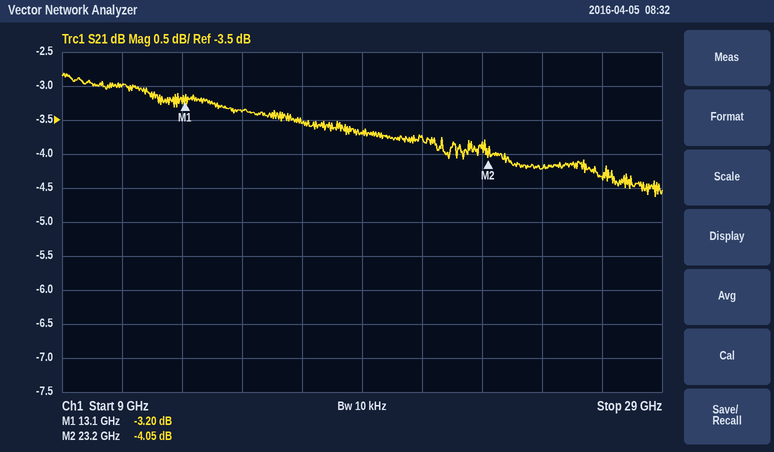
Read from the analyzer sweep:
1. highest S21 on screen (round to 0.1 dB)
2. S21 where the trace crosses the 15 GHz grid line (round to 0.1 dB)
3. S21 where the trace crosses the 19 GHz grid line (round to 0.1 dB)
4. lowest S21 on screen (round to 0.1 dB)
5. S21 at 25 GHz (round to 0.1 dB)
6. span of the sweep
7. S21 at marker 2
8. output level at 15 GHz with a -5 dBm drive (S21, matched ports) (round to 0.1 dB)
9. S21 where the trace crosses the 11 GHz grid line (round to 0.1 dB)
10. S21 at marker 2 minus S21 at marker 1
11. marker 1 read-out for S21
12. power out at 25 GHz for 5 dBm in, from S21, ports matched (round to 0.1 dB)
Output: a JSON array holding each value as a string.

["-2.8 dB", "-3.4 dB", "-3.7 dB", "-4.6 dB", "-4.2 dB", "20 GHz", "-4.05 dB", "-8.4 dBm", "-3.0 dB", "-0.85 dB", "-3.20 dB", "0.8 dBm"]
